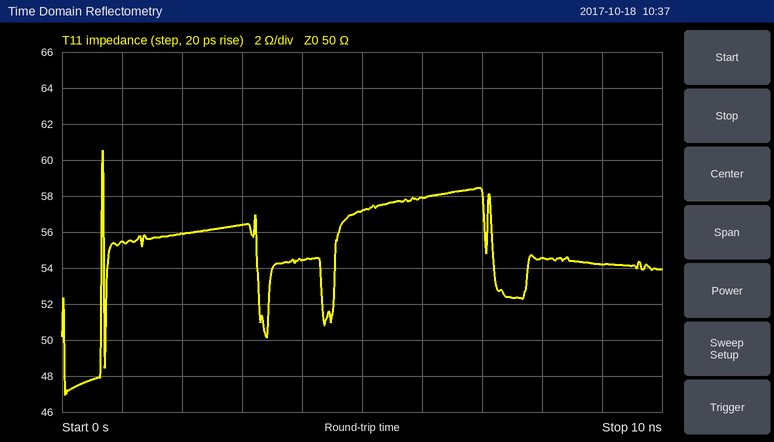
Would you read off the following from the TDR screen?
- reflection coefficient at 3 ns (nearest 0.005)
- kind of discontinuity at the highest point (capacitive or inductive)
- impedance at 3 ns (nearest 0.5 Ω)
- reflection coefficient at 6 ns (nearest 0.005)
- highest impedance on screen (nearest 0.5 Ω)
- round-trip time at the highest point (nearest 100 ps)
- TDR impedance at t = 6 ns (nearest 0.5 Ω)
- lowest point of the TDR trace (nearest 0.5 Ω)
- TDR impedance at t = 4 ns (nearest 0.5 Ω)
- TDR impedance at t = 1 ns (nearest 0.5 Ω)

+0.060
inductive
56.5 Ω
+0.075
60.5 Ω
700 ps
58.0 Ω
47.0 Ω
54.5 Ω
55.5 Ω
